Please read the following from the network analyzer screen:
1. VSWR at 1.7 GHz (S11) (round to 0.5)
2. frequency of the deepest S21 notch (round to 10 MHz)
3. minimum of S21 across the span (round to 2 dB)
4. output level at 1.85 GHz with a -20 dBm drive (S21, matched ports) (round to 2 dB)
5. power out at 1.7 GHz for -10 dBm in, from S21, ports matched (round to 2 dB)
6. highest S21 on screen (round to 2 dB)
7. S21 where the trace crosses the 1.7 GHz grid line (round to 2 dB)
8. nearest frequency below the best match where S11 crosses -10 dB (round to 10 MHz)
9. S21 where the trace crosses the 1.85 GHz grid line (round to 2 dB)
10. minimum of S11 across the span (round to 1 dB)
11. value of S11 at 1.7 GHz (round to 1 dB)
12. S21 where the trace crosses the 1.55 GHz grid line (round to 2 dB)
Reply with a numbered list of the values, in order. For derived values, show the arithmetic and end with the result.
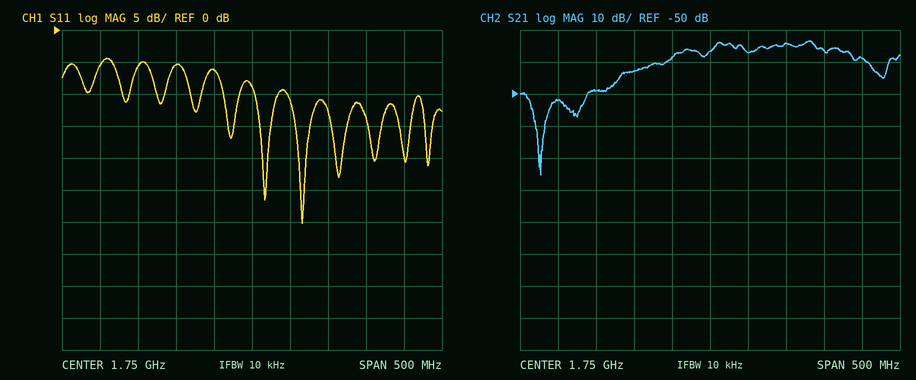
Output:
1. |Γ| = 10^(-6/20) = 0.5012; VSWR = (1 + 0.5012)/(1 − 0.5012) ≈ 3.0
2. 1.53 GHz
3. -76 dB
4. -20 dBm + (-34 dB) = -54 dBm
5. -10 dBm + (-38 dB) = -48 dBm
6. -34 dB
7. -38 dB
8. 1.80 GHz
9. -34 dB
10. -30 dB
11. -6 dB
12. -52 dB
